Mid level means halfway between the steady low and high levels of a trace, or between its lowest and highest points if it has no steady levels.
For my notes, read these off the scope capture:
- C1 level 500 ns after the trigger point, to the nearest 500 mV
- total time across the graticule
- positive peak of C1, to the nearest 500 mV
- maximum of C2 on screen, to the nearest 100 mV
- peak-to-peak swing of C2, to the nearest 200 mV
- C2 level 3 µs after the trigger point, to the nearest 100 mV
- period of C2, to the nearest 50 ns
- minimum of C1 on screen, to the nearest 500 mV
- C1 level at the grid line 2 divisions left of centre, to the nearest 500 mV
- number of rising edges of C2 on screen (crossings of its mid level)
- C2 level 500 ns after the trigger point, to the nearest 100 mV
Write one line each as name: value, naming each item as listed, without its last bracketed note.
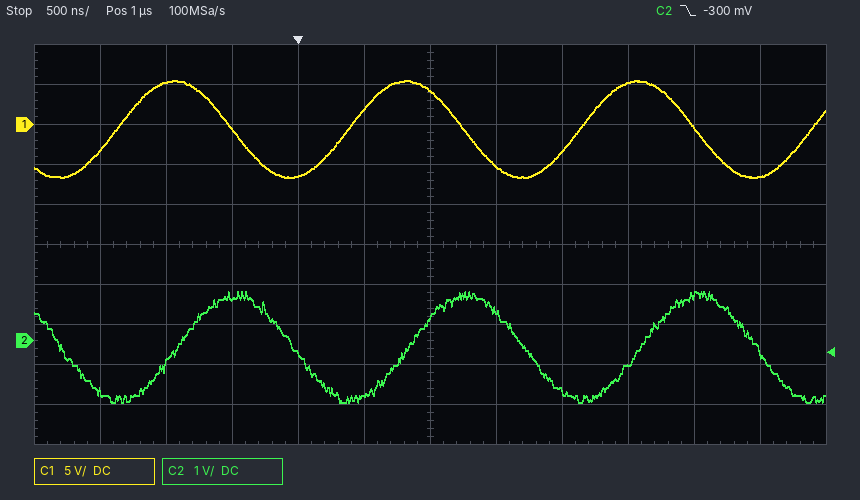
C1 level 500 ns after the trigger point, to the nearest 500 mV: 2.0 V
total time across the graticule: 6 µs
positive peak of C1, to the nearest 500 mV: 5.5 V
maximum of C2 on screen, to the nearest 100 mV: 1.2 V
peak-to-peak swing of C2, to the nearest 200 mV: 2.8 V
C2 level 3 µs after the trigger point, to the nearest 100 mV: 1.1 V
period of C2, to the nearest 50 ns: 1.75 µs
minimum of C1 on screen, to the nearest 500 mV: -6.5 V
C1 level at the grid line 2 divisions left of centre, to the nearest 500 mV: -6.5 V
number of rising edges of C2 on screen: 3
C2 level 500 ns after the trigger point, to the nearest 100 mV: -1.4 V
